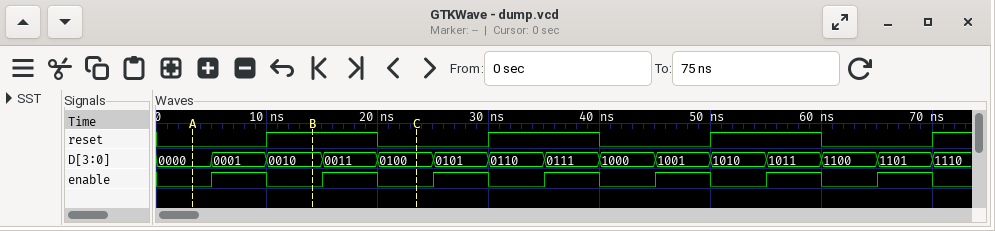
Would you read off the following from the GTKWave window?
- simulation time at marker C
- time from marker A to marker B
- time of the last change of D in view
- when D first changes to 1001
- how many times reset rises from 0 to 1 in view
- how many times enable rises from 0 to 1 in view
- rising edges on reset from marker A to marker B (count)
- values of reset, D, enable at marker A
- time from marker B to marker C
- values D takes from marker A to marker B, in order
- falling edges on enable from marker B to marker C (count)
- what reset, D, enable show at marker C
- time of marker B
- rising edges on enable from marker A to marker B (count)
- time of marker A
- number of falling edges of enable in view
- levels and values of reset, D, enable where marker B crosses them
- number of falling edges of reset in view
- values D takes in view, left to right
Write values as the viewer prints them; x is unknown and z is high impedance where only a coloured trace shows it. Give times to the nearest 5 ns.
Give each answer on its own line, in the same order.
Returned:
25 ns
10 ns
70 ns
45 ns
4
7
1
reset=0, D=0000, enable=0
10 ns
0000, 0001, 0010
1
reset=0, D=0100, enable=0
15 ns
1
5 ns
7
reset=1, D=0010, enable=0
3
0000, 0001, 0010, 0011, 0100, 0101, 0110, 0111, 1000, 1001, 1010, 1011, 1100, 1101, 1110
